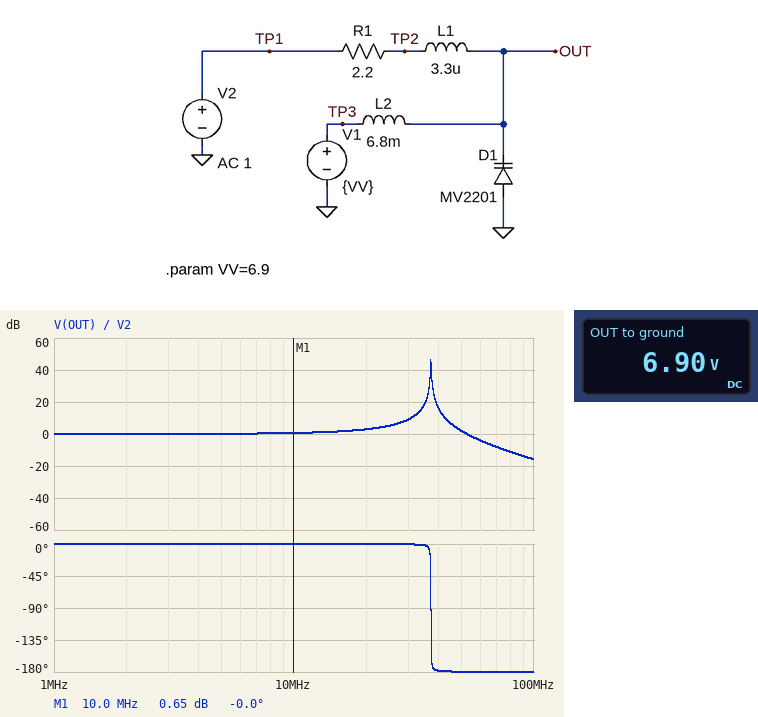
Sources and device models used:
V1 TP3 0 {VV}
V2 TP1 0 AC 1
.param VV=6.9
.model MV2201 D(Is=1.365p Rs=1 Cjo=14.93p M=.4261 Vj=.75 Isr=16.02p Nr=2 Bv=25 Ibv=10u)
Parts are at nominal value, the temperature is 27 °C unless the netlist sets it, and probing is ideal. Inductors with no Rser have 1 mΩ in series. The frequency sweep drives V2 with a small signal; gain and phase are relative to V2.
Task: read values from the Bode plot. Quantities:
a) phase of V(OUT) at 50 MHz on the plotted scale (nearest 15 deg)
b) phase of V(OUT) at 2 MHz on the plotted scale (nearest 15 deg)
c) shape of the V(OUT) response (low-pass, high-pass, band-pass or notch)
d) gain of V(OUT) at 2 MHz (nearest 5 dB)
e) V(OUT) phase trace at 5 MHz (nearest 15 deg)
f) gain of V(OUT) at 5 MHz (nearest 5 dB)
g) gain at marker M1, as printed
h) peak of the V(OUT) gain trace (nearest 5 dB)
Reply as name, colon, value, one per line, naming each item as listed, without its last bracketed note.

phase of V(OUT) at 50 MHz on the plotted scale: -180 deg
phase of V(OUT) at 2 MHz on the plotted scale: 0 deg
shape of the V(OUT) response: low-pass
gain of V(OUT) at 2 MHz: 0 dB
V(OUT) phase trace at 5 MHz: 0 deg
gain of V(OUT) at 5 MHz: 0 dB
gain at marker M1, as printed: 0.65 dB
peak of the V(OUT) gain trace: 45 dB
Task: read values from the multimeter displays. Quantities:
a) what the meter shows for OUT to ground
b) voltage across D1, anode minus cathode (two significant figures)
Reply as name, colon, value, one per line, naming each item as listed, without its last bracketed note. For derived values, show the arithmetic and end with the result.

what the meter shows for OUT to ground: 6.90 V
voltage across D1, anode minus cathode: 0 V - 6.9 V = -6.9 V
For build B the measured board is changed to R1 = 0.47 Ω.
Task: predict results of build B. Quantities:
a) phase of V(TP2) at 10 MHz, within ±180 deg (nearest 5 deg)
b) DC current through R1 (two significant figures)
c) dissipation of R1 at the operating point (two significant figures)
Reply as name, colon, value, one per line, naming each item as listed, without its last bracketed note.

phase of V(TP2) at 10 MHz, within ±180 deg: 0 deg
DC current through R1: 15 A
dissipation of R1 at the operating point: 100 W
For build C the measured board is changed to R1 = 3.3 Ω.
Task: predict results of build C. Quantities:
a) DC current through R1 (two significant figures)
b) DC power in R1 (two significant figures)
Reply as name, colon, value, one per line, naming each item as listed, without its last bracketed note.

DC current through R1: 2.1 A
DC power in R1: 14 W
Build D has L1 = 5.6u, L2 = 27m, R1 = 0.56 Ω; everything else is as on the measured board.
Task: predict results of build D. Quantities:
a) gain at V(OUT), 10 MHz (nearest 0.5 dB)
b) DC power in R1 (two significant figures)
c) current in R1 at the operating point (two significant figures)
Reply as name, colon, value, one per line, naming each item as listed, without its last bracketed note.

gain at V(OUT), 10 MHz: 1.0 dB
DC power in R1: 84 W
current in R1 at the operating point: 12 A
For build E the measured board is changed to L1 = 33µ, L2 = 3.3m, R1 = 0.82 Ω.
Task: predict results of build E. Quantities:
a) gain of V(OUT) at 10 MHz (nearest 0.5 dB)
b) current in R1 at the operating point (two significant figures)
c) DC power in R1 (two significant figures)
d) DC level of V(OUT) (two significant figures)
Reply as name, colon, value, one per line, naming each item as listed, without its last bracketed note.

gain of V(OUT) at 10 MHz: 11.0 dB
current in R1 at the operating point: 8.4 A
DC power in R1: 58 W
DC level of V(OUT): 6.9 V
